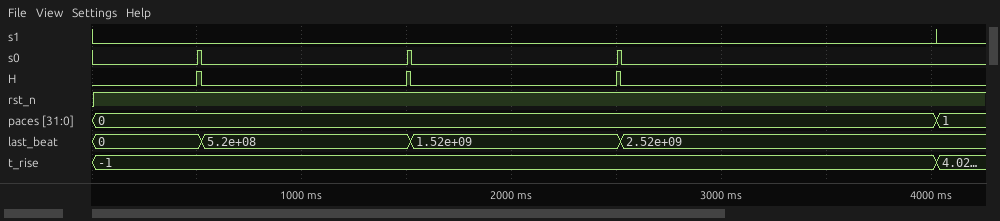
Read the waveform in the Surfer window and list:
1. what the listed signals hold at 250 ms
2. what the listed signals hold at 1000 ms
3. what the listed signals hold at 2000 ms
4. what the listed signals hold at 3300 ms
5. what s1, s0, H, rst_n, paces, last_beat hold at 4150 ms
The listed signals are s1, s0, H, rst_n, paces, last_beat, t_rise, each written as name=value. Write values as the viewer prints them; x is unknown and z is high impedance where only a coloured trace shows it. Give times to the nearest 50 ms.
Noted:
s1=0, s0=0, H=0, rst_n=1, paces=0, last_beat=0, t_rise=-1
s1=0, s0=0, H=0, rst_n=1, paces=0, last_beat=5.2e+08, t_rise=-1
s1=0, s0=0, H=0, rst_n=1, paces=0, last_beat=1.52e+09, t_rise=-1
s1=0, s0=0, H=0, rst_n=1, paces=0, last_beat=2.52e+09, t_rise=-1
s1=0, s0=0, H=0, rst_n=1, paces=1, last_beat=2.52e+09
